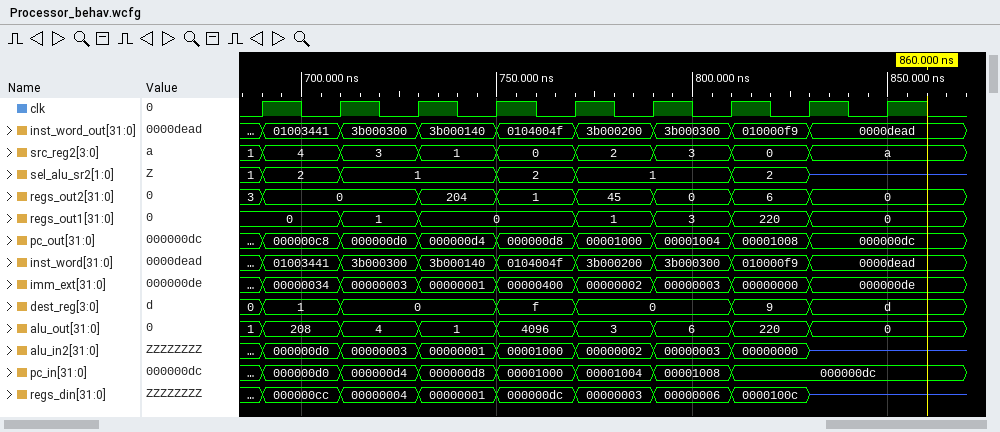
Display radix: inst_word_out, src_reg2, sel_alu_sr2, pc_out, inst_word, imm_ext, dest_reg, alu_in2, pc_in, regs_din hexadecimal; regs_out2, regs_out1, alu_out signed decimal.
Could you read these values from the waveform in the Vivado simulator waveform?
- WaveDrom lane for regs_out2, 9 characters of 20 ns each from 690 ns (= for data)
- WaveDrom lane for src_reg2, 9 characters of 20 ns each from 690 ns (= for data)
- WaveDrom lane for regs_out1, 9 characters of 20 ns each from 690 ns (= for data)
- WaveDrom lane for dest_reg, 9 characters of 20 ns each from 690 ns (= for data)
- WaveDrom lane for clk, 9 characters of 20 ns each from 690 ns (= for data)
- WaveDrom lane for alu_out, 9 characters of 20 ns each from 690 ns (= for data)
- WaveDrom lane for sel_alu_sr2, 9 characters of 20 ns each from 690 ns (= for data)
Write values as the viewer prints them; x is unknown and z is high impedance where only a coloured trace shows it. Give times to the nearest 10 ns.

{name: 'regs_out2', wave: '=.======.', data: '0 204 1 45 0 6 0'}
{name: 'src_reg2', wave: '========.', data: '4 3 1 0 2 3 0 a'}
{name: 'regs_out1', wave: '===.====.', data: '0 1 0 1 3 220 0'}
{name: 'dest_reg', wave: '==.==.==.', data: '1 0 f 0 9 d'}
{name: 'clk', wave: 'p........'}
{name: 'alu_out', wave: '========.', data: '208 4 1 4096 3 6 220 0'}
{name: 'sel_alu_sr2', wave: '==.==.=z.', data: '2 1 2 1 2'}
